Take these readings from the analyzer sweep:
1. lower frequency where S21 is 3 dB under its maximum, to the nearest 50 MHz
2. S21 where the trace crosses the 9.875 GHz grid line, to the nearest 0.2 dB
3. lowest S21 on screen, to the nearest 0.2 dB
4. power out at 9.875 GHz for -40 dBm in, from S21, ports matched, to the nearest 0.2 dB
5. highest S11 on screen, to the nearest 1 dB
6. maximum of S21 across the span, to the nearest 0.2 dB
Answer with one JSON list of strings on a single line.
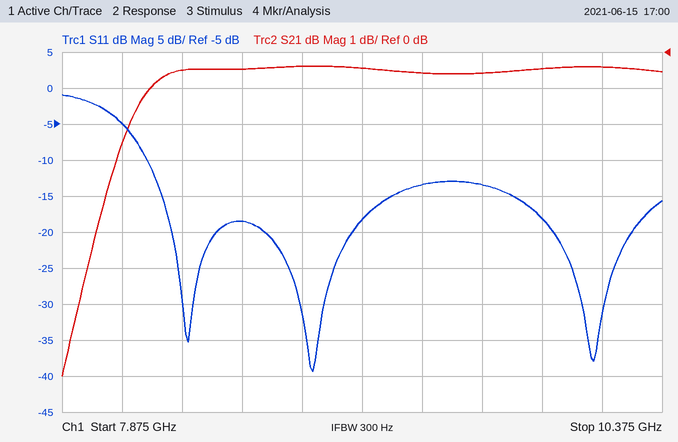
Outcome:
["8.10 GHz", "-0.4 dB", "-9.0 dB", "-40.4 dBm", "-1 dB", "-0.4 dB"]
